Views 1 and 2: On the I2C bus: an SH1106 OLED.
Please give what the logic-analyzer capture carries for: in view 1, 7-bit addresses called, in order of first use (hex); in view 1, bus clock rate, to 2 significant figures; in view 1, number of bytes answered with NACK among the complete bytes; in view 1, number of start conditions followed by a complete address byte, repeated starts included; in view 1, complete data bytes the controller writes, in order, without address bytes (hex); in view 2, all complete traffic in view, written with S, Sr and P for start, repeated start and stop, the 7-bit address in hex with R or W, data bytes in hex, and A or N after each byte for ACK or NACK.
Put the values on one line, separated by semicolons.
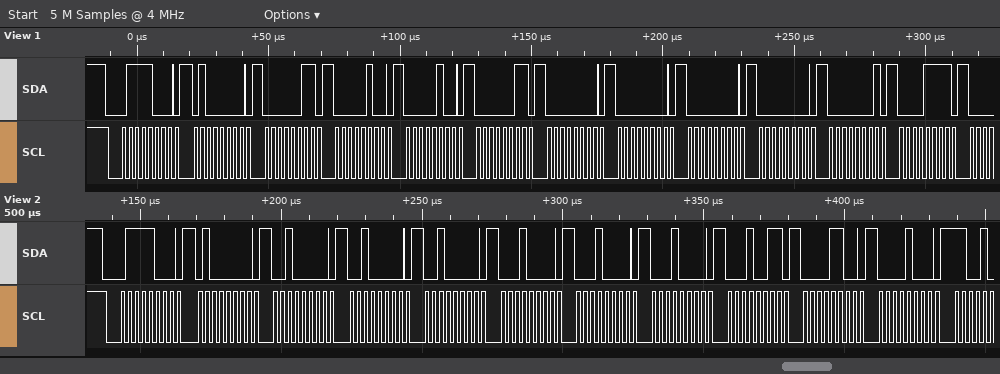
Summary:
0x3C; 400 kHz; 0; 1; 40 03 04 04 03 00 00 00 00 01 0F; S 3CW A 40 A 20 A 20 A 20 A 10 A 10 A 10 A 13 A 0C A 08 A
